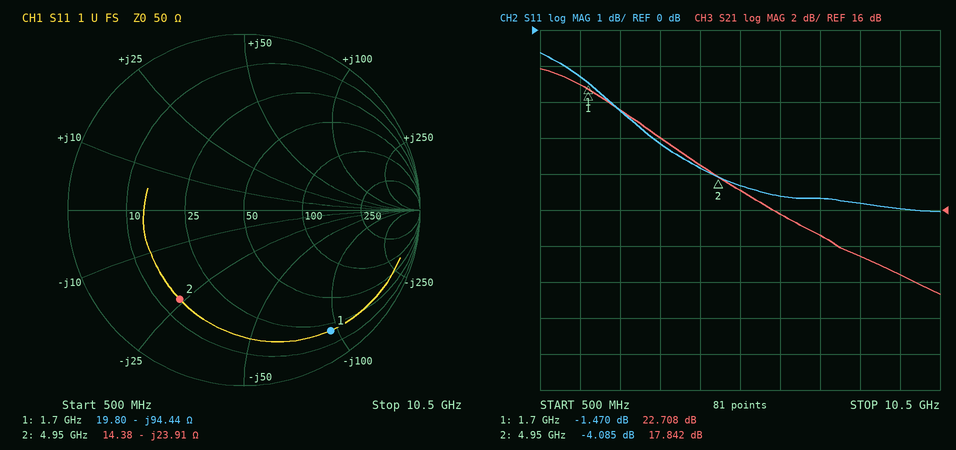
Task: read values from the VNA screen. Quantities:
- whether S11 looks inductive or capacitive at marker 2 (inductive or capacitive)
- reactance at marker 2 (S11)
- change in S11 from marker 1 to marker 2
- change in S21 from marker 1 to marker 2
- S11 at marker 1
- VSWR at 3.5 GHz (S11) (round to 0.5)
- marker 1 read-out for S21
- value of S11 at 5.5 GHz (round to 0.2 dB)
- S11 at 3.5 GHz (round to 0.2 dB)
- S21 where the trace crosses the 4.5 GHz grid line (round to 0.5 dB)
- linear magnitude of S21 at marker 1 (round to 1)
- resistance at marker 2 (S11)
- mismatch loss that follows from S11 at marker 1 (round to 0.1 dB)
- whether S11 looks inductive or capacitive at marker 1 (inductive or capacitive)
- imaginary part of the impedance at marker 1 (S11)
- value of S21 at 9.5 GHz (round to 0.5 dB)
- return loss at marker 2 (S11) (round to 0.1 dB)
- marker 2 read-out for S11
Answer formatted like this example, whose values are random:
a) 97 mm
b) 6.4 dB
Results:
a) capacitive
b) -23.91 Ω
c) -2.615 dB
d) -4.866 dB
e) -1.470 dB
f) 5.5
g) 22.708 dB
h) -4.4 dB
i) -3.2 dB
j) 18.5 dB
k) 14
l) 14.38 Ω
m) 5.4 dB
n) capacitive
o) -94.44 Ω
p) 12.5 dB
q) 4.1 dB
r) -4.085 dB
